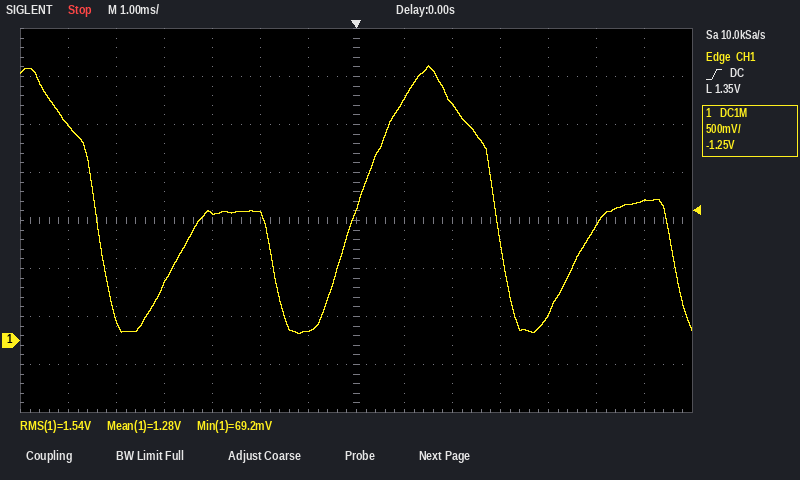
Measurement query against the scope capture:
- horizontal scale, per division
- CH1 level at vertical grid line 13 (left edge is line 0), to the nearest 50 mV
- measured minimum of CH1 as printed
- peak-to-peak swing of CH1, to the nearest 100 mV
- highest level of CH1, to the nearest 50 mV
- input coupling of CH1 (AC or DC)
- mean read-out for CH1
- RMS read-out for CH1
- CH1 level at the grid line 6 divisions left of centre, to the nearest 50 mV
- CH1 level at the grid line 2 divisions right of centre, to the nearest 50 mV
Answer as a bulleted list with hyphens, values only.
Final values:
- 1 ms
- 1.45 V
- 69.2 mV
- 2.80 V
- 2.85 V
- DC
- 1.28 V
- 1.54 V
- 2.25 V
- 2.45 V
